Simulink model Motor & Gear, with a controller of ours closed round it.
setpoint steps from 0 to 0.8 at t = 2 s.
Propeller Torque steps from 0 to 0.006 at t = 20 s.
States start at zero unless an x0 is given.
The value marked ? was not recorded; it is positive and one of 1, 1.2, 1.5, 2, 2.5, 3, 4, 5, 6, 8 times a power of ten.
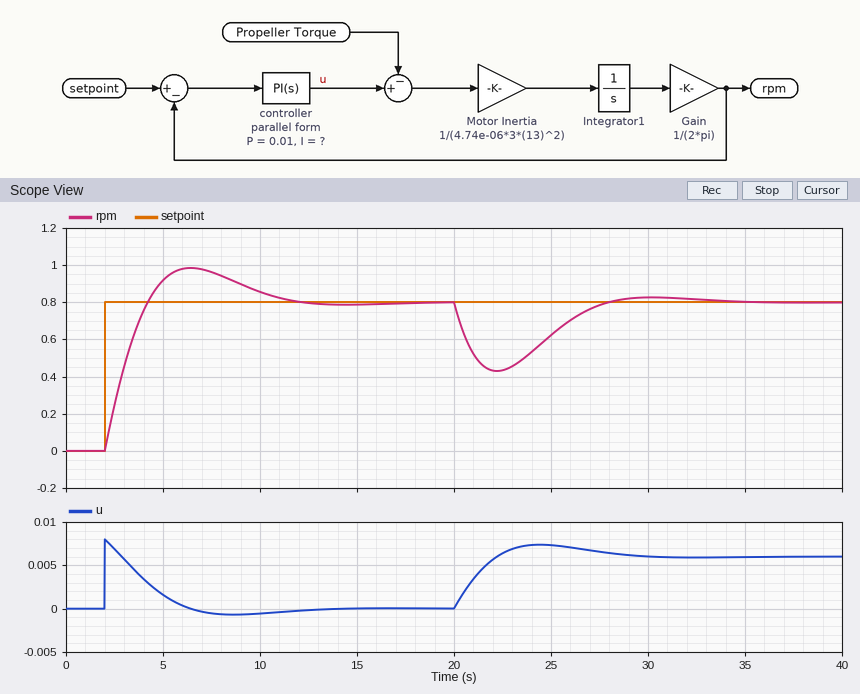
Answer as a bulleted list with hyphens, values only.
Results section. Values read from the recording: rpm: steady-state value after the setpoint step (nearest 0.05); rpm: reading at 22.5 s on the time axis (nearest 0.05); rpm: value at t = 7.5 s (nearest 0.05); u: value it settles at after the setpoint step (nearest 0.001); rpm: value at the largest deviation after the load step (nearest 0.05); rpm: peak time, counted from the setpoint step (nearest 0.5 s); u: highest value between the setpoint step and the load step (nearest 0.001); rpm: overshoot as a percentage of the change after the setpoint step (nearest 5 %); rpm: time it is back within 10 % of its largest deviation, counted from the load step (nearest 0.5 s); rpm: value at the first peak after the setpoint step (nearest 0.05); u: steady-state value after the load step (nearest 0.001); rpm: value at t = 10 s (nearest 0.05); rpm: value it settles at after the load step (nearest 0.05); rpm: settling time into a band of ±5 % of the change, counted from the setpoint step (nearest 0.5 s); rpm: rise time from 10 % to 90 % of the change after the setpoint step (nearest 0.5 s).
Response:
- 0.80
- 0.45
- 0.95
- 0.000
- 0.45
- 4.5 s
- 0.008
- 25 %
- 7.0 s
- 1.00
- 0.006
- 0.85
- 0.80
- 8.5 s
- 1.5 s
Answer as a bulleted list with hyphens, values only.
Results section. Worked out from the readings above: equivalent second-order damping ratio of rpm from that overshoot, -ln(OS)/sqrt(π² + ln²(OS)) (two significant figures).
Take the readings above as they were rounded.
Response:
- 0.40
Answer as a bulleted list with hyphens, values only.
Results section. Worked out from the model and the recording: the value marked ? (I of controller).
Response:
- 0.004
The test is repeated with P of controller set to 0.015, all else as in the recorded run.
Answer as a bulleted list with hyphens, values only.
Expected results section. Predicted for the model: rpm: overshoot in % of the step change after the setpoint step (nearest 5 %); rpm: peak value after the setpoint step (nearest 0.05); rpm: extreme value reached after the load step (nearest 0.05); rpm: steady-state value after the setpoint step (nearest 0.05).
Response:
- 15 %
- 0.90
- 0.50
- 0.80
